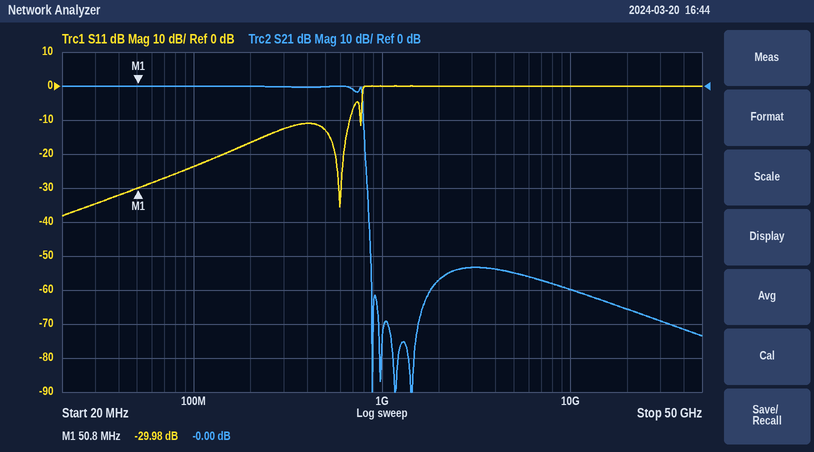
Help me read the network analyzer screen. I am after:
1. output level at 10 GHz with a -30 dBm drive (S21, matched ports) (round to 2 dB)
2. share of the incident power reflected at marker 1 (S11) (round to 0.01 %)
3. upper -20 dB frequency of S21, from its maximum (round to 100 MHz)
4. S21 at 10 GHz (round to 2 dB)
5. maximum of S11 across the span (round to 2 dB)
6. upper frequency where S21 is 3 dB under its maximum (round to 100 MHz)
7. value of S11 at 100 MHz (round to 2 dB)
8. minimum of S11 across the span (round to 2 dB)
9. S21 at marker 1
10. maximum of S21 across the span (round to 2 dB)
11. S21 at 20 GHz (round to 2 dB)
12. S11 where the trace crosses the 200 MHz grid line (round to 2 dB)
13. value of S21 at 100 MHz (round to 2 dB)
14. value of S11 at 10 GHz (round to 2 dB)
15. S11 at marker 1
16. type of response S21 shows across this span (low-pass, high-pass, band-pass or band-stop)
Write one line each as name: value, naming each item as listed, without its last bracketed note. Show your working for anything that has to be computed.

output level at 10 GHz with a -30 dBm drive (S21, matched ports): -30 dBm + (-60 dB) = -90 dBm
share of the incident power reflected at marker 1 (S11): 10^(-29.98/10) ≈ 0.10 %
upper -20 dB frequency of S21, from its maximum: 800 MHz
S21 at 10 GHz: -60 dB
maximum of S11 across the span: 0 dB
upper frequency where S21 is 3 dB under its maximum: 800 MHz
value of S11 at 100 MHz: -24 dB
minimum of S11 across the span: -38 dB
S21 at marker 1: -0.00 dB
maximum of S21 across the span: 0 dB
S21 at 20 GHz: -66 dB
S11 where the trace crosses the 200 MHz grid line: -16 dB
value of S21 at 100 MHz: 0 dB
value of S11 at 10 GHz: 0 dB
S11 at marker 1: -29.98 dB
type of response S21 shows across this span: low-pass
